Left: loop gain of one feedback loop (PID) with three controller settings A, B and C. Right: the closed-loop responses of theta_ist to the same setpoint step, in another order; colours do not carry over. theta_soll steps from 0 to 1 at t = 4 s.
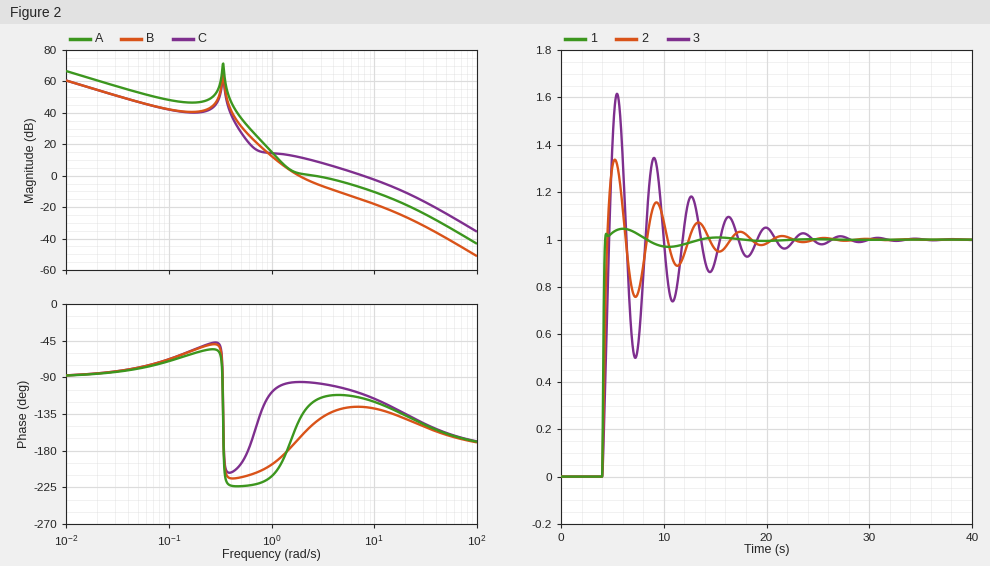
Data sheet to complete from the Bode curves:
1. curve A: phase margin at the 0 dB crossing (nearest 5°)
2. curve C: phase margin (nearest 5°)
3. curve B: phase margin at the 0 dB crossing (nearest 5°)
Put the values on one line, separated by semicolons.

60°; 70°; 15°
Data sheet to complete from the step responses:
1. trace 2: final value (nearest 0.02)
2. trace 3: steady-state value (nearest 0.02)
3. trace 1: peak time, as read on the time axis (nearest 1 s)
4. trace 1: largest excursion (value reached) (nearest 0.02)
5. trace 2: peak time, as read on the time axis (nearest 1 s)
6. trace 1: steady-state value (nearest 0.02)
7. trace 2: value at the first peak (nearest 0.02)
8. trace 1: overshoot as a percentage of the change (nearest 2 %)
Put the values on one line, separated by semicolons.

1.00; 1.00; 6 s; 1.04; 5 s; 1.00; 1.34; 4 %
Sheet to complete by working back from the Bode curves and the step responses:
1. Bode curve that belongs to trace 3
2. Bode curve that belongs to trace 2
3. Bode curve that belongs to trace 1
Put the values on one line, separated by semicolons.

B; A; C
